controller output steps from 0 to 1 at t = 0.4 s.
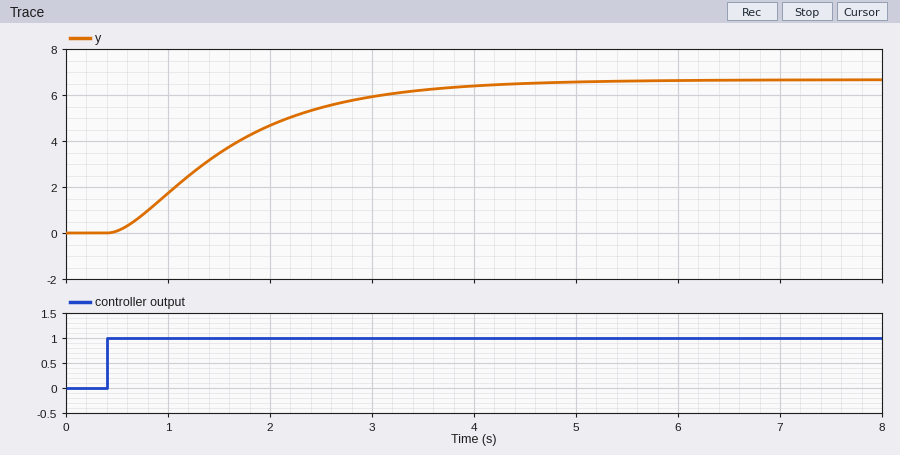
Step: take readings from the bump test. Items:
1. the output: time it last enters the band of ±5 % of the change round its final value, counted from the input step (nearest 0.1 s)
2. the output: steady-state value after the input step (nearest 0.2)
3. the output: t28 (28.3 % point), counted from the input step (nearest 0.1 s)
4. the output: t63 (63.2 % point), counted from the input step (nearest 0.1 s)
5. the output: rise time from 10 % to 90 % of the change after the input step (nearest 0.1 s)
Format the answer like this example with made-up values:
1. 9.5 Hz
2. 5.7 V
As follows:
1. 3.4 s
2. 6.6
3. 0.6 s
4. 1.4 s
5. 2.4 s
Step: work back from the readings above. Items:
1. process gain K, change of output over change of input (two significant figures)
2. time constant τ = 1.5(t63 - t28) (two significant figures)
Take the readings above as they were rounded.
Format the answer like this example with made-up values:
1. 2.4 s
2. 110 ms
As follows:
1. 6.6
2. 1.2 s
